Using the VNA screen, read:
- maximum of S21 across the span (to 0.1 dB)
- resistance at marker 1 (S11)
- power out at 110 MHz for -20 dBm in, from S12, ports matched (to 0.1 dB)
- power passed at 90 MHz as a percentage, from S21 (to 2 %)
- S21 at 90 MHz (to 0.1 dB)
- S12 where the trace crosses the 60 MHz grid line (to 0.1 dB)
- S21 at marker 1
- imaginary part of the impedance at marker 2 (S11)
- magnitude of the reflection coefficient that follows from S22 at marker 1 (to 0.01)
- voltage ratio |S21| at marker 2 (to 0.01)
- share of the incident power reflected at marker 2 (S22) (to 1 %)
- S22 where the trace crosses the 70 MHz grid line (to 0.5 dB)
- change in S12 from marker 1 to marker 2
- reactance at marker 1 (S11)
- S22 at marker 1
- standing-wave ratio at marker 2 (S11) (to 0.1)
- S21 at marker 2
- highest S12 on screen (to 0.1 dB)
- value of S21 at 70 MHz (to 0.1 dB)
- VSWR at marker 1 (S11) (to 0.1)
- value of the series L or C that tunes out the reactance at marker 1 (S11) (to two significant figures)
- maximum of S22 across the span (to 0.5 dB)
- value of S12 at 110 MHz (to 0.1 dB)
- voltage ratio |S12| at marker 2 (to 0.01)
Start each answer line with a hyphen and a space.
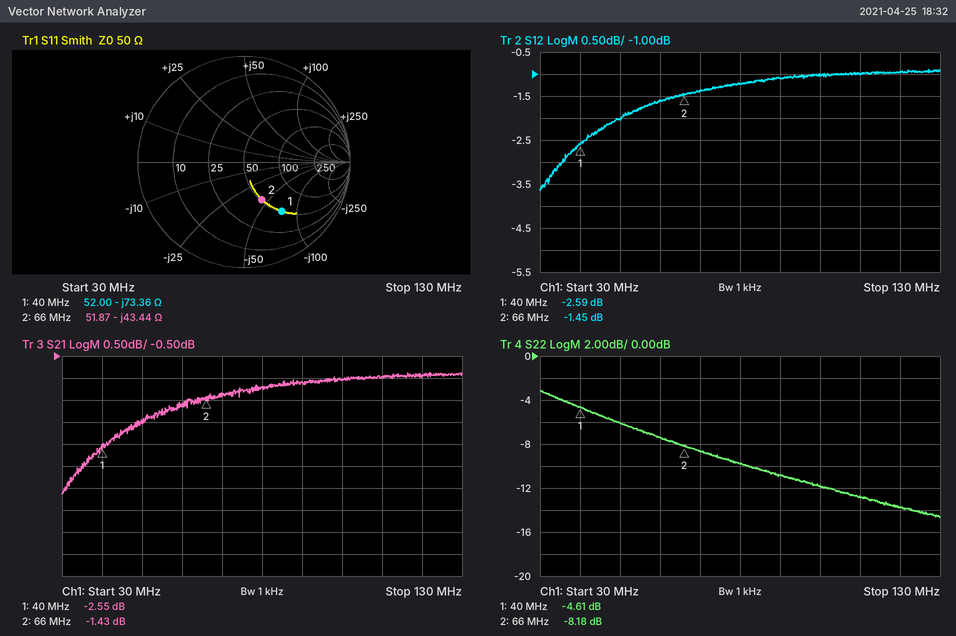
- -0.9 dB
- 52.00 Ω
- -21.0 dBm
- 78 %
- -1.1 dB
- -1.6 dB
- -2.55 dB
- -43.44 Ω
- 0.59
- 0.85
- 15 %
- -8.5 dB
- 1.14 dB
- -73.36 Ω
- -4.61 dB
- 2.3
- -1.43 dB
- -0.9 dB
- -1.4 dB
- 3.8
- 290 nH
- -3.0 dB
- -1.0 dB
- 0.85
